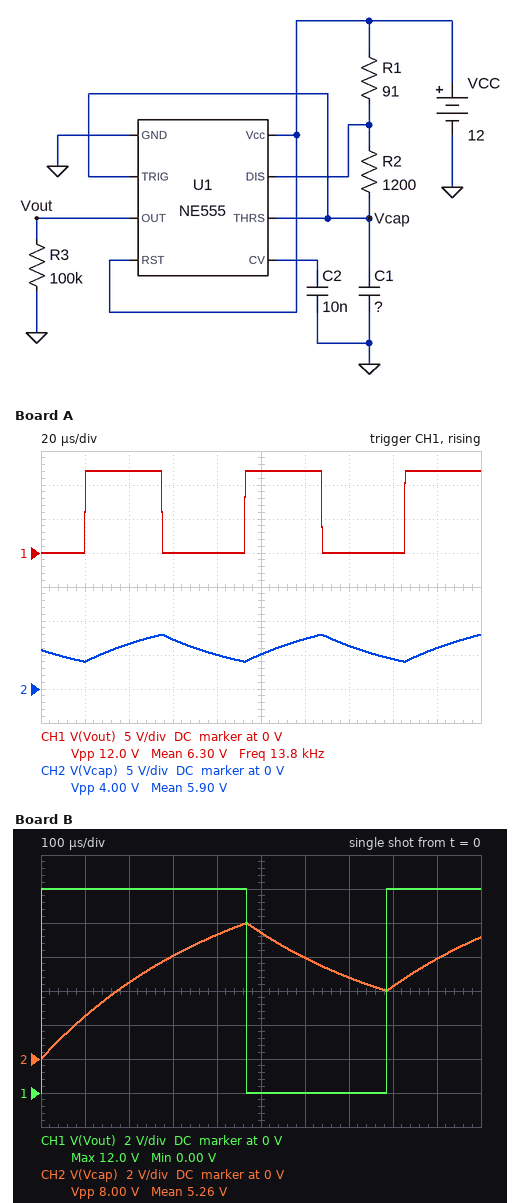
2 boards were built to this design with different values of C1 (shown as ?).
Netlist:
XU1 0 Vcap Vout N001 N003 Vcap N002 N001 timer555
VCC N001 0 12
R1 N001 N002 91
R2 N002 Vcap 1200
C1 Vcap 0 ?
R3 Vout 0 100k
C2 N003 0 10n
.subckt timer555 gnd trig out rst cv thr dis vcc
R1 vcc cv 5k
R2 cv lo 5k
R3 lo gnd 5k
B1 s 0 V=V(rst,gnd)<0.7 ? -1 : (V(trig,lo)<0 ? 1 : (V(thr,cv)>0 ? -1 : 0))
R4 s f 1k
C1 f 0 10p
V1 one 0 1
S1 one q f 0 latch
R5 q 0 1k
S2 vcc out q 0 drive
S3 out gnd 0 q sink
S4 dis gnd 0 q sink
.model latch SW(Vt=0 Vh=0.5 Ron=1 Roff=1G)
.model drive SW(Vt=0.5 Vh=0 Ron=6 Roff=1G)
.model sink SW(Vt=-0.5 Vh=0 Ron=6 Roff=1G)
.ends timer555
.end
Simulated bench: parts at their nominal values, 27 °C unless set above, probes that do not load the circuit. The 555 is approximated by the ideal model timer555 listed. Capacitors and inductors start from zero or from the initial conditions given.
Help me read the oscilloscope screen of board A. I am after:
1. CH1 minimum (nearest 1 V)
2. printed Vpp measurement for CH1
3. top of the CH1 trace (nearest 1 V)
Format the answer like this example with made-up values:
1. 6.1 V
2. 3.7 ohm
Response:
1. 0 V
2. 12.0 V
3. 12 V
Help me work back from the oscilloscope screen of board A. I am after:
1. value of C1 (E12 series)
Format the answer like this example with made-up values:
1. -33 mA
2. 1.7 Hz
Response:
1. 39 nF
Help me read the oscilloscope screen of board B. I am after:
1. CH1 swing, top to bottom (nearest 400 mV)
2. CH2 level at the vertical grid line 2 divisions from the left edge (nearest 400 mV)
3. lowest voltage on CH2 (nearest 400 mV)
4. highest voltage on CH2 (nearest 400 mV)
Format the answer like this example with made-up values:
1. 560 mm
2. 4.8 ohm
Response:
1. 12.0 V
2. 4.4 V
3. 0 V
4. 8.0 V
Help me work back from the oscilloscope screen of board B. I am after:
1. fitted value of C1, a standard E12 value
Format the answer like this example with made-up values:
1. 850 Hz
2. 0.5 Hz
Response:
1. 330 nF
